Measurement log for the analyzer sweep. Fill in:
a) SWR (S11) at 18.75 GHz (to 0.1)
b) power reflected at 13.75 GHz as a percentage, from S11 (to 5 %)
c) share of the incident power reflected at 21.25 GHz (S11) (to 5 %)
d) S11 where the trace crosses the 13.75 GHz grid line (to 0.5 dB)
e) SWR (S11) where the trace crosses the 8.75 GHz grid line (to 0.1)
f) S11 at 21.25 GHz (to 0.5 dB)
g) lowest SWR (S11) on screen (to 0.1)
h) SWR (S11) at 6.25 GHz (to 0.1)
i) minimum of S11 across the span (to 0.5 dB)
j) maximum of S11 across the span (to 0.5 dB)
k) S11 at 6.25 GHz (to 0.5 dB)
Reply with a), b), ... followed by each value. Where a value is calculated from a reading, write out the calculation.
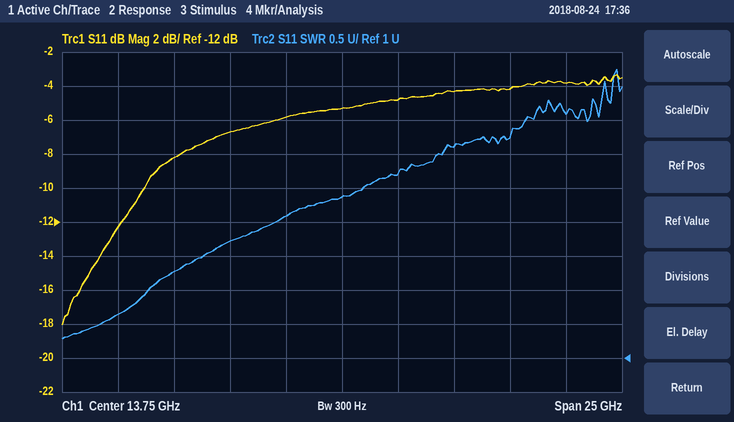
a) 4.1
b) 10^(-5.5/10) ≈ 28.2 %, so 30 % to the nearest 5 %
c) 10^(-4/10) ≈ 40 %
d) -5.5 dB
e) 2.7
f) -4.0 dB
g) 1.3
h) 2.3
i) -18.0 dB
j) -3.5 dB
k) -8.0 dB
